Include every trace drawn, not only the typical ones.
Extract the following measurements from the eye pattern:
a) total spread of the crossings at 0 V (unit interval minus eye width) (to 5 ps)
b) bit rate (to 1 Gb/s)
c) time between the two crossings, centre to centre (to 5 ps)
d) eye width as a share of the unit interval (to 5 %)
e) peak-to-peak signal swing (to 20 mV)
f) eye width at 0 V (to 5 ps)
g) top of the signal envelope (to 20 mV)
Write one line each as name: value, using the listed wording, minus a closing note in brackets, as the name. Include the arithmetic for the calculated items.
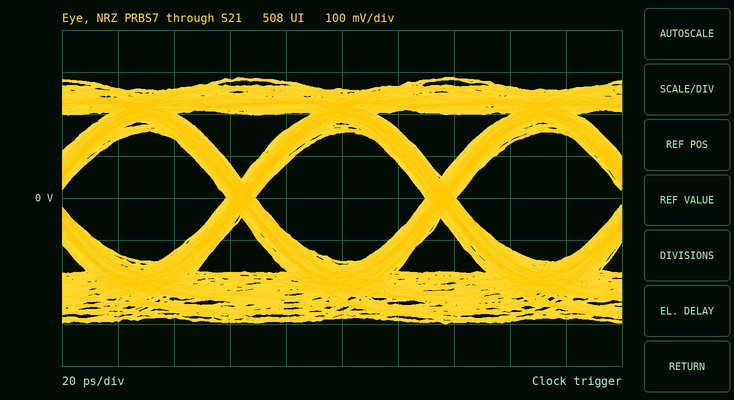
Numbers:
total spread of the crossings at 0 V (unit interval minus eye width): 10 ps
bit rate: 14 Gb/s
time between the two crossings, centre to centre: 70 ps
eye width as a share of the unit interval: 60 ps / 70 ps ≈ 85.7 %, so 85 % to the nearest 5 %
peak-to-peak signal swing: 580 mV
eye width at 0 V: 60 ps
top of the signal envelope: 280 mV
